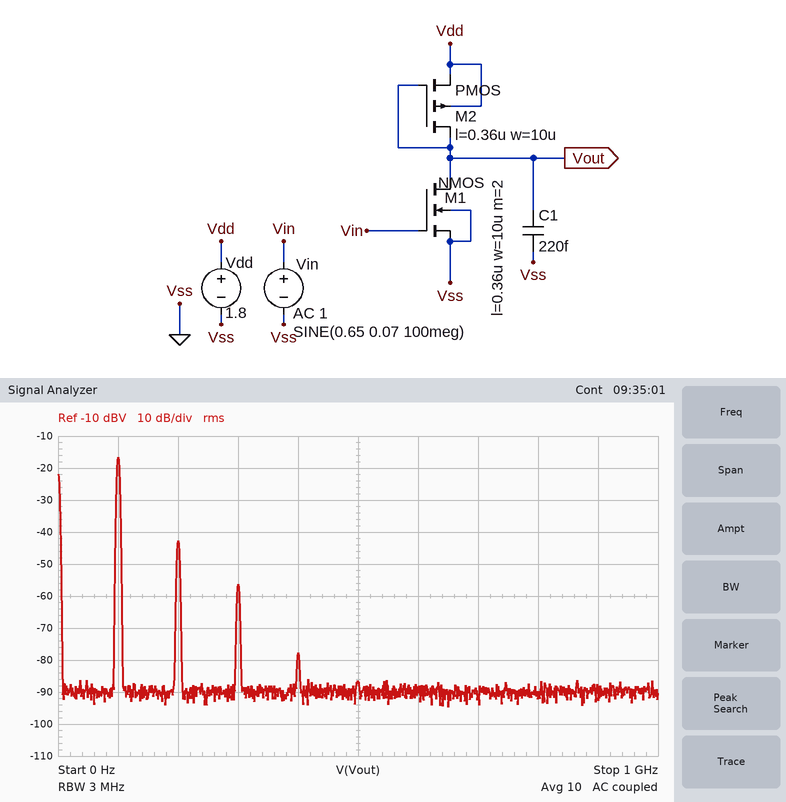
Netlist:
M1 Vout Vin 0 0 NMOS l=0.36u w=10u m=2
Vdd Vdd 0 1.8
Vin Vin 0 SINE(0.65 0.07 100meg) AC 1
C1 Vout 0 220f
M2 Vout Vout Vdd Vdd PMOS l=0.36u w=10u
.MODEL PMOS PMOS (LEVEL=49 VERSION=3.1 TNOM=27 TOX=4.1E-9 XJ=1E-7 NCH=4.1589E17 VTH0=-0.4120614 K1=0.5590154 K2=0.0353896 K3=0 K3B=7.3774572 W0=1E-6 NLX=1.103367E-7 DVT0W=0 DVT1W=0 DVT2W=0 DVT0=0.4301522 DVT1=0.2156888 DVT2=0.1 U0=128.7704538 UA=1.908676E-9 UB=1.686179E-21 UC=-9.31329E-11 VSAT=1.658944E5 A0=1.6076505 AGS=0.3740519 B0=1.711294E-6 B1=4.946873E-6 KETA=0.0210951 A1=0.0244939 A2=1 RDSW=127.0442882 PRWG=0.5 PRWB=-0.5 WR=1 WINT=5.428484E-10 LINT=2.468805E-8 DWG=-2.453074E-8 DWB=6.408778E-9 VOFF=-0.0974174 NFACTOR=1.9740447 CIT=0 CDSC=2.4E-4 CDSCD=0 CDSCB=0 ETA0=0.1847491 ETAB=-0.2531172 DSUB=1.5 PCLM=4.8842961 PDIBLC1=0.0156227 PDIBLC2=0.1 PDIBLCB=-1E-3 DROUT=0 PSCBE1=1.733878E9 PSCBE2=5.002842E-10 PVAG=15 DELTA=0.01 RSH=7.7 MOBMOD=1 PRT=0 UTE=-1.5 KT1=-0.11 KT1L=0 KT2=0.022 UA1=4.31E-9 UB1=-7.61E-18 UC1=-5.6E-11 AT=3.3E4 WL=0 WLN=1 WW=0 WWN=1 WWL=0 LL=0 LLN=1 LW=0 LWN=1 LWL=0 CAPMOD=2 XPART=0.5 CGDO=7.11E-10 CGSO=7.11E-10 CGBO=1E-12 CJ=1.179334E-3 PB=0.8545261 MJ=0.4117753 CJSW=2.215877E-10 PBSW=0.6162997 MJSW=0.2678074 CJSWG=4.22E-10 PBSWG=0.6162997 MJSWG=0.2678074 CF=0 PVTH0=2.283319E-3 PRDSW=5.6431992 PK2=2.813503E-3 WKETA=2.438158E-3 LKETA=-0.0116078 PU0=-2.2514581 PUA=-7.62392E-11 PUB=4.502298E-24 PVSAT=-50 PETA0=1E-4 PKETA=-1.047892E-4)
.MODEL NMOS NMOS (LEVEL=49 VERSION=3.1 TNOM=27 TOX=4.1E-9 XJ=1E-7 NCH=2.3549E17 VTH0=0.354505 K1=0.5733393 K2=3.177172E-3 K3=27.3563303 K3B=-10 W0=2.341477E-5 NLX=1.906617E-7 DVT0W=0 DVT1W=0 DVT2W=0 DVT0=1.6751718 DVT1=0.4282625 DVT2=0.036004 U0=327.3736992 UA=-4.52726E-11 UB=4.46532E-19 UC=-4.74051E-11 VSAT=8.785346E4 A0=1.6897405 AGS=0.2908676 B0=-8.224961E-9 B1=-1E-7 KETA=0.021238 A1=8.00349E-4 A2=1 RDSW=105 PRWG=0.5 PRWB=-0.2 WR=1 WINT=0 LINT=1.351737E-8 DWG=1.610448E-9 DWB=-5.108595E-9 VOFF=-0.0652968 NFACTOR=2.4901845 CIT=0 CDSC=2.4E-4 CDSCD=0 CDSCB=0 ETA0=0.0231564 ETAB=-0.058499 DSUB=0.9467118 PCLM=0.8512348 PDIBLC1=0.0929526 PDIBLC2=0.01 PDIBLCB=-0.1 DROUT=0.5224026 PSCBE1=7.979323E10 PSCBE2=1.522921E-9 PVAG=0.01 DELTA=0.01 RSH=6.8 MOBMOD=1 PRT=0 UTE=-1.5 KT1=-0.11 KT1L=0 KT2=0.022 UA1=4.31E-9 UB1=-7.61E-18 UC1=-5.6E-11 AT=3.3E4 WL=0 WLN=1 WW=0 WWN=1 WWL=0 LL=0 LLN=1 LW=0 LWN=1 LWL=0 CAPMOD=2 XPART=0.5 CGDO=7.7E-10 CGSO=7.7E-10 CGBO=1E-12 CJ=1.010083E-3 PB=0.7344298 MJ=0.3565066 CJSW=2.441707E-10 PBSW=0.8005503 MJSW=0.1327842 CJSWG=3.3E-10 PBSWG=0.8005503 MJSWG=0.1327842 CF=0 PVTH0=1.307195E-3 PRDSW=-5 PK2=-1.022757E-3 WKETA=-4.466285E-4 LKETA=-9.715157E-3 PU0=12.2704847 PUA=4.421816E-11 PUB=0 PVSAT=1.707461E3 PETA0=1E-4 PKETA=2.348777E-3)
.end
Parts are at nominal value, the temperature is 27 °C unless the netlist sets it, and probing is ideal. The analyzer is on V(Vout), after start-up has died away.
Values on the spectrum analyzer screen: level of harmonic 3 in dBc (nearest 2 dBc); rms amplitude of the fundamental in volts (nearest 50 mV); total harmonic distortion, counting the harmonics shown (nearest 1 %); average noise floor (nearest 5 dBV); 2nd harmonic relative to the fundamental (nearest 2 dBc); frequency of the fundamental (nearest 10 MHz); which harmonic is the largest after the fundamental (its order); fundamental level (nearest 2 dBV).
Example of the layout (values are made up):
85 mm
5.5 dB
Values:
-40 dBc
150 mV
5 %
-90 dBV
-26 dBc
100 MHz
2
-16 dBV
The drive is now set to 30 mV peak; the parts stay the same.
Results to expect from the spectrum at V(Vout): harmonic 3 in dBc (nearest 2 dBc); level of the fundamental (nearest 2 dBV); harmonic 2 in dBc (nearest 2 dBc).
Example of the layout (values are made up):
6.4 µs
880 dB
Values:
-54 dBc
-24 dBV
-34 dBc
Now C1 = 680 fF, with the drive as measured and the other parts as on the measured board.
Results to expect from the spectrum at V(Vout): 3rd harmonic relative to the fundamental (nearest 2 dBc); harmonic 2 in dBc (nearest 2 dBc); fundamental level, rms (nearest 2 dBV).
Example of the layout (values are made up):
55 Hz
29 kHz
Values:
-42 dBc
-22 dBc
-18 dBV
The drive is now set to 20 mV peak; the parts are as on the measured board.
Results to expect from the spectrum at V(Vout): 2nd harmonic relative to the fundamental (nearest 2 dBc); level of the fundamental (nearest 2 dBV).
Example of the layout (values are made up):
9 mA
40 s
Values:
-38 dBc
-28 dBV
